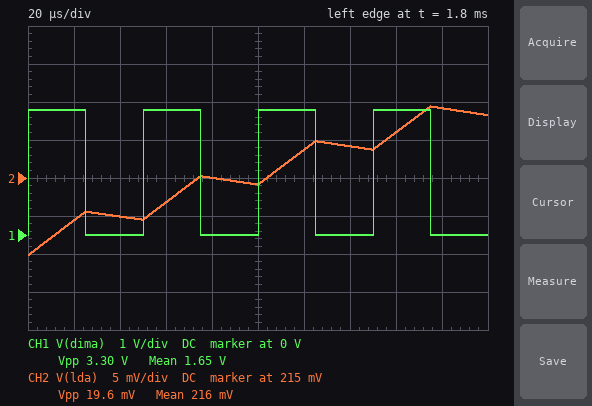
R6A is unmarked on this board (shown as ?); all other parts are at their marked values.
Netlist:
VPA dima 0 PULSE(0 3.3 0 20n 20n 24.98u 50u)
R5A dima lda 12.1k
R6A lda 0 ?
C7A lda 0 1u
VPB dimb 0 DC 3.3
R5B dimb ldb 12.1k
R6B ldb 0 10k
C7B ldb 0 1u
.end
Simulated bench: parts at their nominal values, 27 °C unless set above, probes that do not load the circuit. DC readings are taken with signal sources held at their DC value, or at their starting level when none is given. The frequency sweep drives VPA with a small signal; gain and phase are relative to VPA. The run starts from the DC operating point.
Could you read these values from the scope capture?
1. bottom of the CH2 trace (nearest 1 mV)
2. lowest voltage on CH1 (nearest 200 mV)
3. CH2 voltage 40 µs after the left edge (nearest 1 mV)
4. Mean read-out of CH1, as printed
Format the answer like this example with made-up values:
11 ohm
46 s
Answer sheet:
205 mV
0 V
210 mV
1.65 V
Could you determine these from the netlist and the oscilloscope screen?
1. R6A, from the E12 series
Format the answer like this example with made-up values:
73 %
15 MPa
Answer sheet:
8.2 kΩ
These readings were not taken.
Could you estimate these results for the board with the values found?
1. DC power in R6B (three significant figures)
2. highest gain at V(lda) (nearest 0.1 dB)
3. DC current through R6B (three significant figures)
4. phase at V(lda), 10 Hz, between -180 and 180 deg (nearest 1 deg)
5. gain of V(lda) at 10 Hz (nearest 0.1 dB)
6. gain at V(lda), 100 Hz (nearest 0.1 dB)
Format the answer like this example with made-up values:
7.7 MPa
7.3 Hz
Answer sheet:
223 µW
-7.9 dB
149 µA
-17 deg
-8.3 dB
-18.1 dB
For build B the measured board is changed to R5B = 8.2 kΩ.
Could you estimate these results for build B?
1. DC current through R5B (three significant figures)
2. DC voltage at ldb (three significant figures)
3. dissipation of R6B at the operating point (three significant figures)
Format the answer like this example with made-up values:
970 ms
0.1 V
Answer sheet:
181 µA
1.81 V
329 µW
